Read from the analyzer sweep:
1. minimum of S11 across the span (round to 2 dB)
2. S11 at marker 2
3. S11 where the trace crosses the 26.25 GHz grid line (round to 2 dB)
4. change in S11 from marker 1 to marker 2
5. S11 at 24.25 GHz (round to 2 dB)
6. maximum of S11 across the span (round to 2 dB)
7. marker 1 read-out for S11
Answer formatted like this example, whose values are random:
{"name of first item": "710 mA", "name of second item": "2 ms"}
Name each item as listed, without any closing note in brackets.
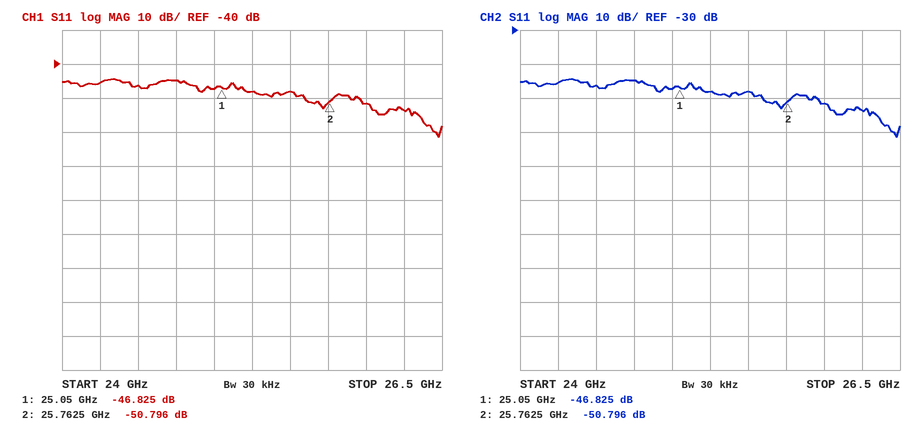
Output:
{"minimum of S11 across the span": "-62 dB", "S11 at marker 2": "-50.796 dB", "S11 where the trace crosses the 26.25 GHz grid line": "-54 dB", "change in S11 from marker 1 to marker 2": "-3.971 dB", "S11 at 24.25 GHz": "-46 dB", "maximum of S11 across the span": "-44 dB", "marker 1 read-out for S11": "-46.825 dB"}
